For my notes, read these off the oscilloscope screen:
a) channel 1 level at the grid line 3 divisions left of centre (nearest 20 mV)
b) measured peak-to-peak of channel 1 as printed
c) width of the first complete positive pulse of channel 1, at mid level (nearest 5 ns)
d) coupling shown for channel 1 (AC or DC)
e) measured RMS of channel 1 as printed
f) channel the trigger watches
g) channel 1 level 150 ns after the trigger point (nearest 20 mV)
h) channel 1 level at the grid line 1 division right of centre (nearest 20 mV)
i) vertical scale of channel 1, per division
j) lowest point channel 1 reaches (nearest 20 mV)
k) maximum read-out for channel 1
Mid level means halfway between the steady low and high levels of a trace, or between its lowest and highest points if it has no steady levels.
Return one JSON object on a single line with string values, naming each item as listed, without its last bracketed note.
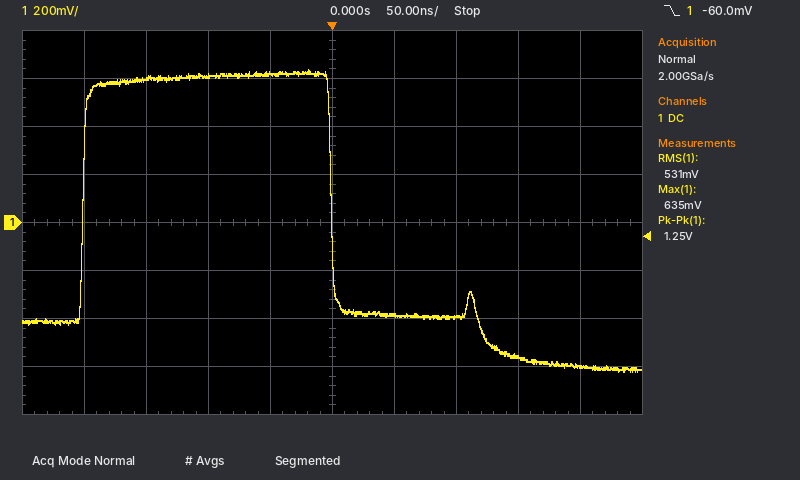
{"channel 1 level at the grid line 3 divisions left of centre": "600 mV", "measured peak-to-peak of channel 1 as printed": "1.25 V", "width of the first complete positive pulse of channel 1, at mid level": "200 ns", "coupling shown for channel 1": "DC", "measured RMS of channel 1 as printed": "531 mV", "channel the trigger watches": "channel 1", "channel 1 level 150 ns after the trigger point": "-560 mV", "channel 1 level at the grid line 1 division right of centre": "-380 mV", "vertical scale of channel 1, per division": "200 mV", "lowest point channel 1 reaches": "-620 mV", "maximum read-out for channel 1": "635 mV"}
